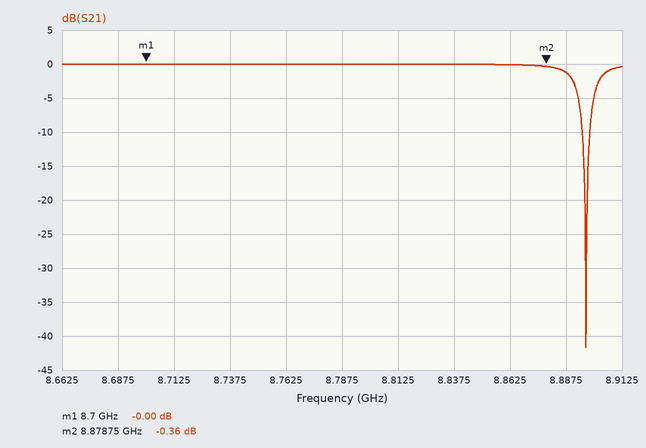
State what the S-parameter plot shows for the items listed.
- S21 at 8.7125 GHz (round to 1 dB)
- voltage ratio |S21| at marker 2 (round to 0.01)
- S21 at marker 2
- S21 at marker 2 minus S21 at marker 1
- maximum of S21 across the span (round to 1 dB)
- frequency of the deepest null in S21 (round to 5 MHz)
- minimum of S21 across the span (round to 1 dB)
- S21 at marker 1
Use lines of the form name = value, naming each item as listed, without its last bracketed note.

S21 at 8.7125 GHz = 0 dB
voltage ratio |S21| at marker 2 = 0.96
S21 at marker 2 = -0.36 dB
S21 at marker 2 minus S21 at marker 1 = -0.36 dB
maximum of S21 across the span = 0 dB
frequency of the deepest null in S21 = 8.895 GHz
minimum of S21 across the span = -42 dB
S21 at marker 1 = -0.00 dB
